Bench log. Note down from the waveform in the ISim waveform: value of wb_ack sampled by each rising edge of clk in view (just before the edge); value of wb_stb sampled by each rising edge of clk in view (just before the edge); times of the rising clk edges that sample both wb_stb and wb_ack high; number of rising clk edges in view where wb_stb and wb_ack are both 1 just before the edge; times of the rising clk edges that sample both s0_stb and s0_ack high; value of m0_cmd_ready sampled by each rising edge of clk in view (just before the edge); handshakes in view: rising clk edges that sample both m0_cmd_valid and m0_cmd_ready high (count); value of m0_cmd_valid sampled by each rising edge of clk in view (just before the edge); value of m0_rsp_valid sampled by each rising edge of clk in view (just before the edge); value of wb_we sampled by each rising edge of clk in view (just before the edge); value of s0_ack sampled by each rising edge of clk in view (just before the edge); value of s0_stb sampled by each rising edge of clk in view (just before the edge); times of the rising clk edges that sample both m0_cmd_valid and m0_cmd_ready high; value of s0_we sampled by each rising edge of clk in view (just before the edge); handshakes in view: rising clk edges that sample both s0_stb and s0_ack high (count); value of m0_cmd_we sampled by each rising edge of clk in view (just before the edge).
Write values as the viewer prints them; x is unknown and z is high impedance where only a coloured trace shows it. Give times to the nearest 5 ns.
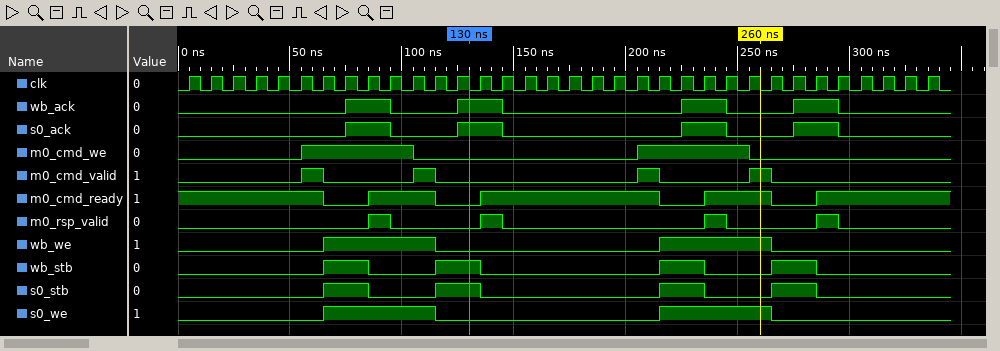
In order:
0 0 0 0 0 0 0 0 1 1 0 0 0 1 1 0 0 0 0 0 0 0 0 1 1 0 0 0 1 1 0 0 0 0
0 0 0 0 0 0 0 1 1 0 0 0 1 1 0 0 0 0 0 0 0 0 1 1 0 0 0 1 1 0 0 0 0 0
85 ns, 135 ns, 235 ns, 285 ns
4
85 ns, 135 ns, 235 ns, 285 ns
1 1 1 1 1 1 1 0 0 1 1 1 0 0 1 1 1 1 1 1 1 1 0 0 1 1 1 0 0 1 1 1 1 1
4
0 0 0 0 0 0 1 0 0 0 0 1 0 0 0 0 0 0 0 0 0 1 0 0 0 0 1 0 0 0 0 0 0 0
0 0 0 0 0 0 0 0 0 1 0 0 0 0 1 0 0 0 0 0 0 0 0 0 1 0 0 0 0 1 0 0 0 0
0 0 0 0 0 0 0 1 1 1 1 1 0 0 0 0 0 0 0 0 0 0 1 1 1 1 1 0 0 0 0 0 0 0
0 0 0 0 0 0 0 0 1 1 0 0 0 1 1 0 0 0 0 0 0 0 0 1 1 0 0 0 1 1 0 0 0 0
0 0 0 0 0 0 0 1 1 0 0 0 1 1 0 0 0 0 0 0 0 0 1 1 0 0 0 1 1 0 0 0 0 0
65 ns, 115 ns, 215 ns, 265 ns
0 0 0 0 0 0 0 1 1 1 1 1 0 0 0 0 0 0 0 0 0 0 1 1 1 1 1 0 0 0 0 0 0 0
4
0 0 0 0 0 0 1 1 1 1 1 0 0 0 0 0 0 0 0 0 0 1 1 1 1 1 0 0 0 0 0 0 0 0
